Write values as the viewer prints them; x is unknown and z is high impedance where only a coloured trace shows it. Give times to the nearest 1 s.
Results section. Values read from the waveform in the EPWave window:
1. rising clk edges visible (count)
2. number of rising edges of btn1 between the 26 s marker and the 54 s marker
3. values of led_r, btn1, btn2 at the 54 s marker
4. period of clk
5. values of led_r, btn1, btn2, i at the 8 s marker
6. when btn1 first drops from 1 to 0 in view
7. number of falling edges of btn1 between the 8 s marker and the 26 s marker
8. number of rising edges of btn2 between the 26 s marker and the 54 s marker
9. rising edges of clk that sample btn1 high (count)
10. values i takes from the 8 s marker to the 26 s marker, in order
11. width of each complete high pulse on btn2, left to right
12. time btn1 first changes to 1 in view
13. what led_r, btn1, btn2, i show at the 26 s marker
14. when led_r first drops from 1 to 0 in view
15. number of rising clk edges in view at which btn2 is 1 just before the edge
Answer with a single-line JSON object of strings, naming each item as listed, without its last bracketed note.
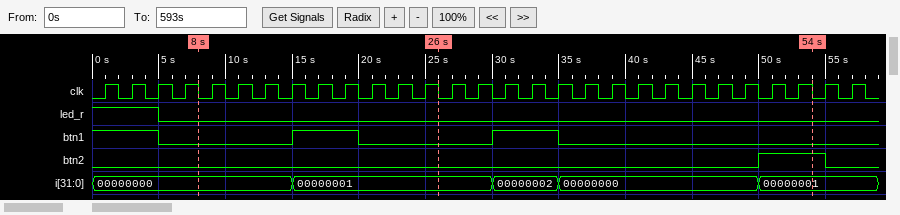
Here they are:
{"rising clk edges visible": "29", "number of rising edges of btn1 between the 26 s marker and the 54 s marker": "1", "values of led_r, btn1, btn2 at the 54 s marker": "led_r=0, btn1=0, btn2=1", "period of clk": "2 s", "values of led_r, btn1, btn2, i at the 8 s marker": "led_r=0, btn1=0, btn2=0, i=00000000", "when btn1 first drops from 1 to 0 in view": "5 s", "number of falling edges of btn1 between the 8 s marker and the 26 s marker": "1", "number of rising edges of btn2 between the 26 s marker and the 54 s marker": "1", "rising edges of clk that sample btn1 high": "8", "values i takes from the 8 s marker to the 26 s marker, in order": "00000000, 00000001", "width of each complete high pulse on btn2, left to right": "5 s", "time btn1 first changes to 1 in view": "15 s", "what led_r, btn1, btn2, i show at the 26 s marker": "led_r=0, btn1=0, btn2=0, i=00000001", "when led_r first drops from 1 to 0 in view": "5 s", "number of rising clk edges in view at which btn2 is 1 just before the edge": "3"}
